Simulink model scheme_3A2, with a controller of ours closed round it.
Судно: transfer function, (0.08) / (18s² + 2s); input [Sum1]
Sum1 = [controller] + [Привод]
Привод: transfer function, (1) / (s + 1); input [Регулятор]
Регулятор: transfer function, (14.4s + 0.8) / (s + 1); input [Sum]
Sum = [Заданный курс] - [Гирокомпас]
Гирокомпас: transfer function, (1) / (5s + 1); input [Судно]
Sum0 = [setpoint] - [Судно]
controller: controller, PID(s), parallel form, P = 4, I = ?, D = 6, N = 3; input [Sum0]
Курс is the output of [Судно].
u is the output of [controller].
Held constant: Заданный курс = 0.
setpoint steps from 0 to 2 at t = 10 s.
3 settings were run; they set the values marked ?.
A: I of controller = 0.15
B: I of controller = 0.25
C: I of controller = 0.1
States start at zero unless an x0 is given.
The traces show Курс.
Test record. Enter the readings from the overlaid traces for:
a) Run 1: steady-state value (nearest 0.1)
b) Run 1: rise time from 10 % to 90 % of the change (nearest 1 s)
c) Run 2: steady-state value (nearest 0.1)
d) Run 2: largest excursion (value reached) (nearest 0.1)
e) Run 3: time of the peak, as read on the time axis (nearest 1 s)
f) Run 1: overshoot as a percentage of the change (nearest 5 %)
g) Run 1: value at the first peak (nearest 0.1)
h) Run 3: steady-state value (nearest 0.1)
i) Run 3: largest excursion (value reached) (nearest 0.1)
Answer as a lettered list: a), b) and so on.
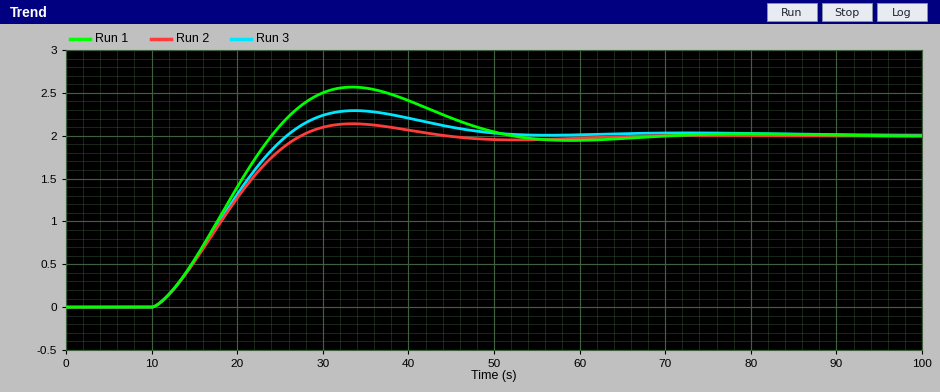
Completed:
a) 2.0
b) 10 s
c) 2.0
d) 2.1
e) 34 s
f) 30 %
g) 2.6
h) 2.0
i) 2.3
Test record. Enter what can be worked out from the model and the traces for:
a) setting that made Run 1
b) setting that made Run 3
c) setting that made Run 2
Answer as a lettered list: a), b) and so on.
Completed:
a) B
b) A
c) C
